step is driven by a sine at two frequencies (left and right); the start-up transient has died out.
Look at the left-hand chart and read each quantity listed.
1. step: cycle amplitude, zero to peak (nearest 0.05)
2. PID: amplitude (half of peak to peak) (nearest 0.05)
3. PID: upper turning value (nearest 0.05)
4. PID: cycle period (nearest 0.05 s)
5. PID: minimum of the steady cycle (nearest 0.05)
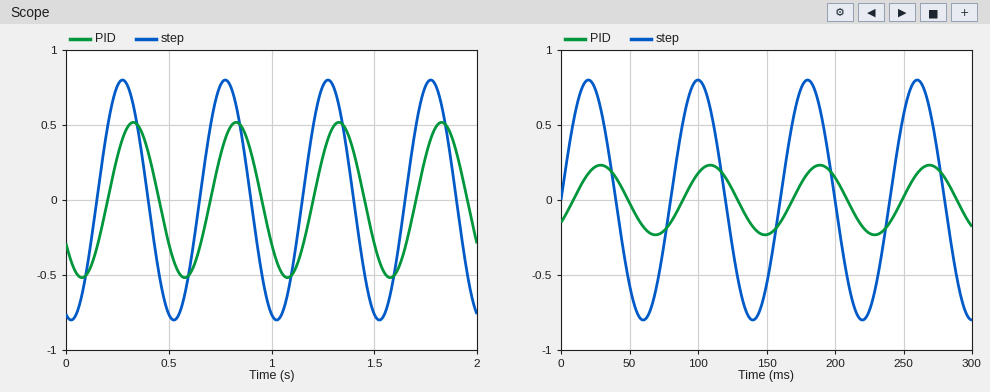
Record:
0.80
0.50
0.50
0.50 s
-0.50
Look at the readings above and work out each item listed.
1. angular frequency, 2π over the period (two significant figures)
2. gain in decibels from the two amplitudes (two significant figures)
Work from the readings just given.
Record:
13 rad/s
-4.1 dB
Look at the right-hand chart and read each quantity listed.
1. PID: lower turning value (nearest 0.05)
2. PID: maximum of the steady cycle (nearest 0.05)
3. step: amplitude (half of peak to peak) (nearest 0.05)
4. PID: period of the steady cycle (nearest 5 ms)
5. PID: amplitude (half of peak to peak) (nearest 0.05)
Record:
-0.25
0.25
0.80
80 ms
0.25
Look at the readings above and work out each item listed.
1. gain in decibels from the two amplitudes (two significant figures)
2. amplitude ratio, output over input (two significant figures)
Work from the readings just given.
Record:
-10 dB
0.31
